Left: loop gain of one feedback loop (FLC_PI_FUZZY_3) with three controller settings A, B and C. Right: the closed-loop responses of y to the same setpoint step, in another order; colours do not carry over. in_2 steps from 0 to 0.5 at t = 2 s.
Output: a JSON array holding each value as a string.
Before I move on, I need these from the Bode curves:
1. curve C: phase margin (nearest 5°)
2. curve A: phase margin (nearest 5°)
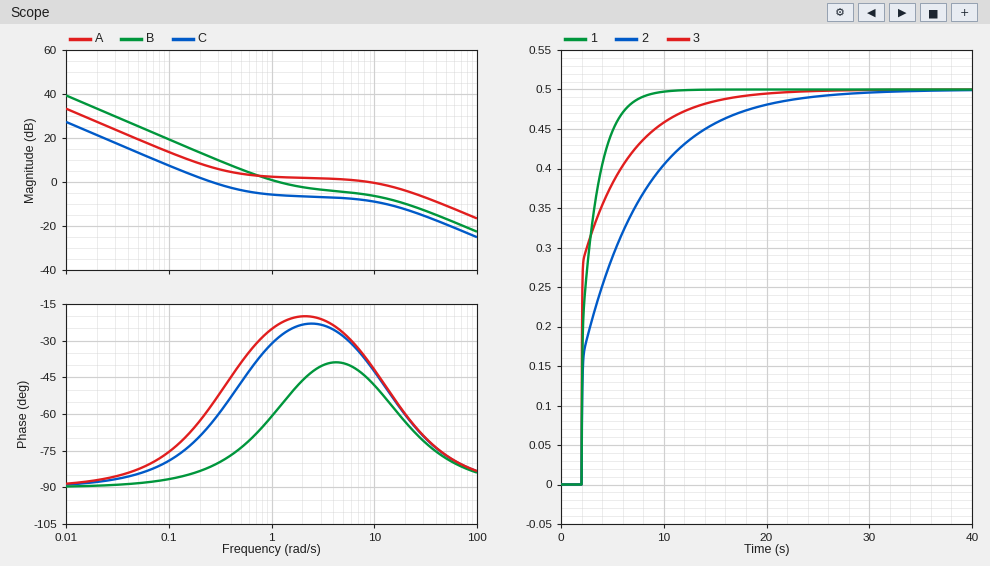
["115°", "140°"]
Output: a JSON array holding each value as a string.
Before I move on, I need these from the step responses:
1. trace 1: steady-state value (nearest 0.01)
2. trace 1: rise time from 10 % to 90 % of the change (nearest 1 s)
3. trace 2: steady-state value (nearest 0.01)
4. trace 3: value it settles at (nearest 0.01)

["0.50", "3 s", "0.50", "0.50"]
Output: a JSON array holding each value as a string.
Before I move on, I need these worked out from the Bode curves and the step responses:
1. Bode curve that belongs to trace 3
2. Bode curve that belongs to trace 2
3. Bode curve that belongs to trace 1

["A", "C", "B"]
